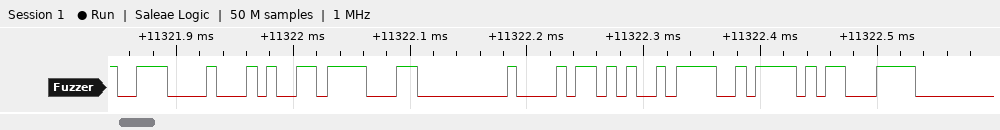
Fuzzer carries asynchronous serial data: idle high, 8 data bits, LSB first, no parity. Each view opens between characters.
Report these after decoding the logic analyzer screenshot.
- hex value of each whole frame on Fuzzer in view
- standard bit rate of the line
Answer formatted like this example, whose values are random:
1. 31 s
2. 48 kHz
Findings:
1. 0E, 94, 8F, 00, 68, E9, 7A, E3
2. 115200 baud
